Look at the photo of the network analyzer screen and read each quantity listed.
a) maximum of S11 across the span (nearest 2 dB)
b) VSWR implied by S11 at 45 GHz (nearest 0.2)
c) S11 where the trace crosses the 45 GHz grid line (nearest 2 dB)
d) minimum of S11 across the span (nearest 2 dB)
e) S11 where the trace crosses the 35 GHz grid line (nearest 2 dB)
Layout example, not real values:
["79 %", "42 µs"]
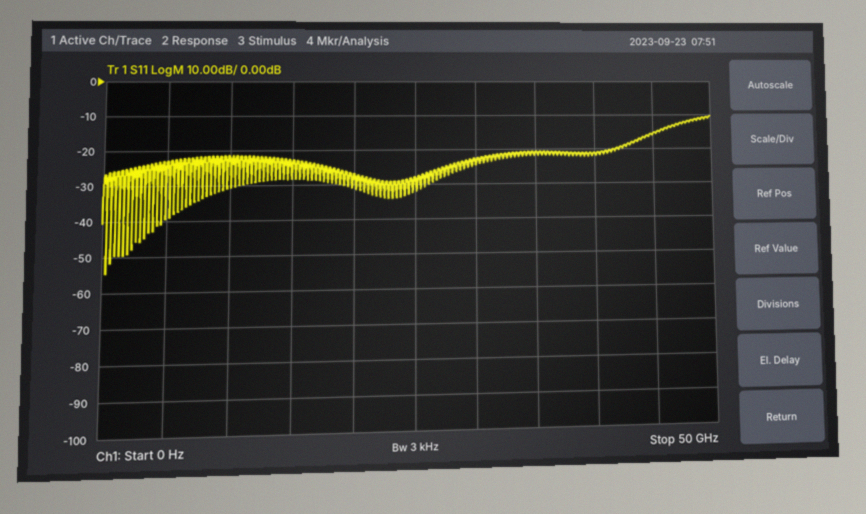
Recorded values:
["-10 dB", "1.4", "-16 dB", "-54 dB", "-22 dB"]
